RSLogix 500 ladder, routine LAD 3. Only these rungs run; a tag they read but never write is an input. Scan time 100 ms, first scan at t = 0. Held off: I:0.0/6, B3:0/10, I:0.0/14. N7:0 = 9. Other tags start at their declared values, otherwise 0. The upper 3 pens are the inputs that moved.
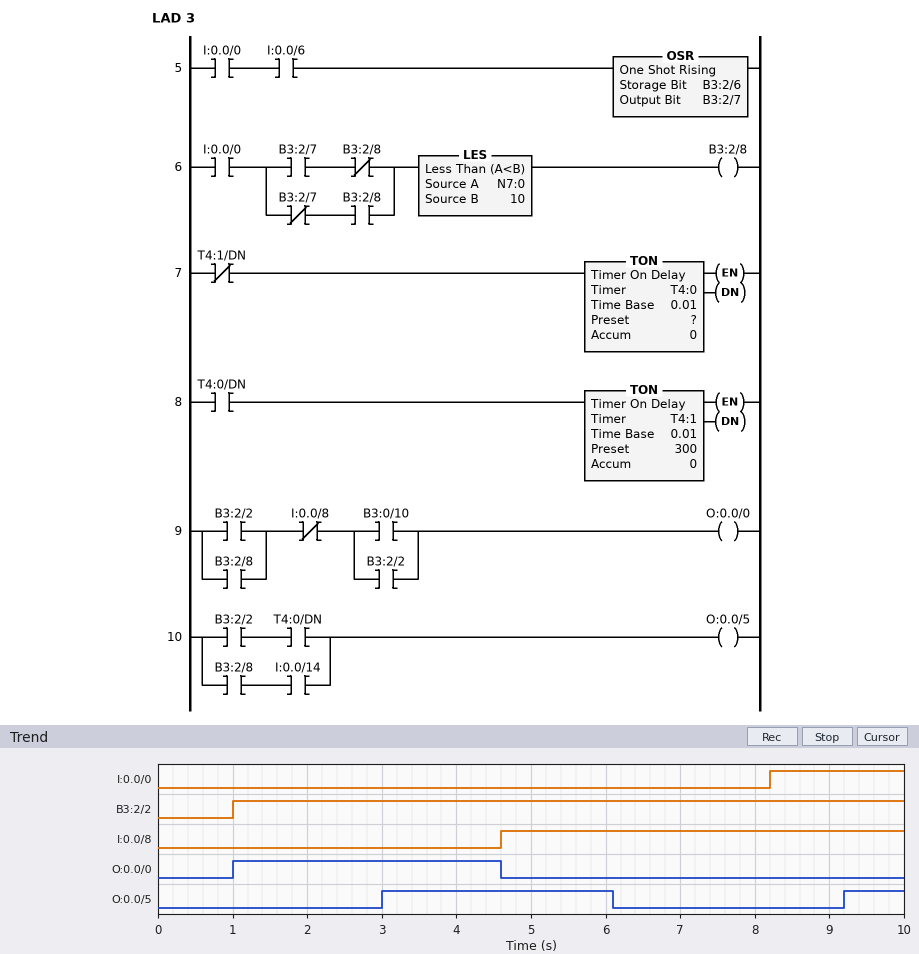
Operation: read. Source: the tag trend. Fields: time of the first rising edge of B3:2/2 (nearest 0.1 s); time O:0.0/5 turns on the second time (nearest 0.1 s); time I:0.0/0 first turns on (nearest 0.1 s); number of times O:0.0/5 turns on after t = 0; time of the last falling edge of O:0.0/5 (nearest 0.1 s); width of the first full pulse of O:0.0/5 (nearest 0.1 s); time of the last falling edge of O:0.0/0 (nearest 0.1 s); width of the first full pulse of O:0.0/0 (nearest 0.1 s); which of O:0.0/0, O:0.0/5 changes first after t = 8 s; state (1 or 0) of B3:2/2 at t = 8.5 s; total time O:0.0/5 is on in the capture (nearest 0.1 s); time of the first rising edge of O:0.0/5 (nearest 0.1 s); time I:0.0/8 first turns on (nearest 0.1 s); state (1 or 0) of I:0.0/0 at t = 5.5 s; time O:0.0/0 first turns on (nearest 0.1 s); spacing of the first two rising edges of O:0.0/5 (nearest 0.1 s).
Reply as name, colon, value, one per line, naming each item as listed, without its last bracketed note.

time of the first rising edge of B3:2/2: 1.0 s
time O:0.0/5 turns on the second time: 9.2 s
time I:0.0/0 first turns on: 8.2 s
number of times O:0.0/5 turns on after t = 0: 2
time of the last falling edge of O:0.0/5: 6.1 s
width of the first full pulse of O:0.0/5: 3.1 s
time of the last falling edge of O:0.0/0: 4.6 s
width of the first full pulse of O:0.0/0: 3.6 s
which of O:0.0/0, O:0.0/5 changes first after t = 8 s: O:0.0/5
state (1 or 0) of B3:2/2 at t = 8.5 s: 1
total time O:0.0/5 is on in the capture: 3.9 s
time of the first rising edge of O:0.0/5: 3.0 s
time I:0.0/8 first turns on: 4.6 s
state (1 or 0) of I:0.0/0 at t = 5.5 s: 0
time O:0.0/0 first turns on: 1.0 s
spacing of the first two rising edges of O:0.0/5: 6.2 s
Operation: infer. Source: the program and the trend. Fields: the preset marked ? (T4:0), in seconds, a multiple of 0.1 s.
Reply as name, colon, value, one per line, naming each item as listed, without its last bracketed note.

the preset marked ? (T4:0), in seconds, a multiple of 0.1 s: 3.0 s
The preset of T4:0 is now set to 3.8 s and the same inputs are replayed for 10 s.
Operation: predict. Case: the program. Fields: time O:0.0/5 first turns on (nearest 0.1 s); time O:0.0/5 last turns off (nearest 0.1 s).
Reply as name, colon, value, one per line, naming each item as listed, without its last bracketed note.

time O:0.0/5 first turns on: 3.8 s
time O:0.0/5 last turns off: 6.9 s
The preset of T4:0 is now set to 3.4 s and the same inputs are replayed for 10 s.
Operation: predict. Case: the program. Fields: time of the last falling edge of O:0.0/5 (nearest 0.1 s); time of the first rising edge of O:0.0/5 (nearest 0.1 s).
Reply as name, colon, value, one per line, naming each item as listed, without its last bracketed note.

time of the last falling edge of O:0.0/5: 6.5 s
time of the first rising edge of O:0.0/5: 3.4 s
